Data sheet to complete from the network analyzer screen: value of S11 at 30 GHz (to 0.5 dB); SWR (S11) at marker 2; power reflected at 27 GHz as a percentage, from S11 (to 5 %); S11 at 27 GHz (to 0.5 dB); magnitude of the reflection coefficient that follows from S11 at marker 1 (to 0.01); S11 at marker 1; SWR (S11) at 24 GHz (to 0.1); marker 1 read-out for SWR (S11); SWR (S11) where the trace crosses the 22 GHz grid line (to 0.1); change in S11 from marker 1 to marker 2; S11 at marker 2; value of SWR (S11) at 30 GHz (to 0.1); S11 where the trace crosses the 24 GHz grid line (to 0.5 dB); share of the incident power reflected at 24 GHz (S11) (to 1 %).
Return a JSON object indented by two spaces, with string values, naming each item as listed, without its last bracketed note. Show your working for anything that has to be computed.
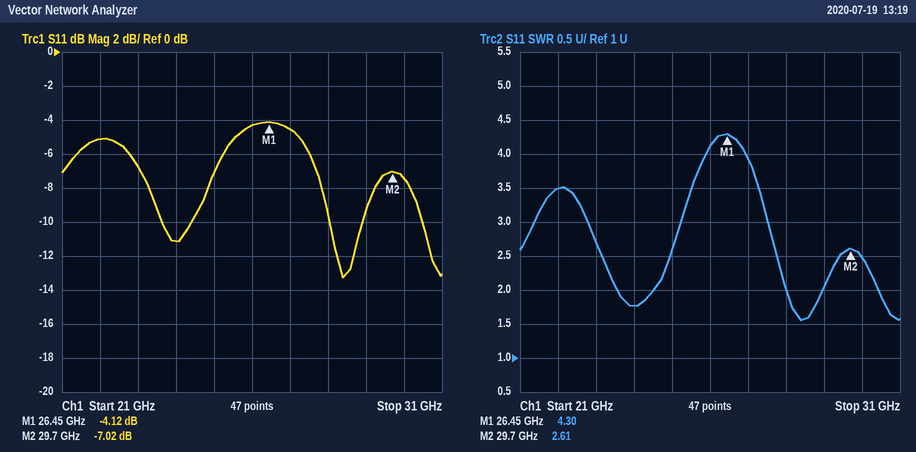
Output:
{
  "value of S11 at 30 GHz": "-7.5 dB",
  "SWR (S11) at marker 2": "2.61",
  "power reflected at 27 GHz as a percentage, from S11": "10^(-4.5/10) ≈ 35 %",
  "S11 at 27 GHz": "-4.5 dB",
  "magnitude of the reflection coefficient that follows from S11 at marker 1": "10^(-4.12/20) ≈ 0.62",
  "S11 at marker 1": "-4.12 dB",
  "SWR (S11) at 24 GHz": "1.8",
  "marker 1 read-out for SWR": "4.30",
  "SWR (S11) where the trace crosses the 22 GHz grid line": "3.5",
  "change in S11 from marker 1 to marker 2": "-7.02 − (-4.12) = -2.90 dB",
  "S11 at marker 2": "-7.02 dB",
  "value of SWR (S11) at 30 GHz": "2.5",
  "S11 where the trace crosses the 24 GHz grid line": "-11.0 dB",
  "share of the incident power reflected at 24 GHz (S11)": "10^(-11/10) ≈ 8 %"
}
